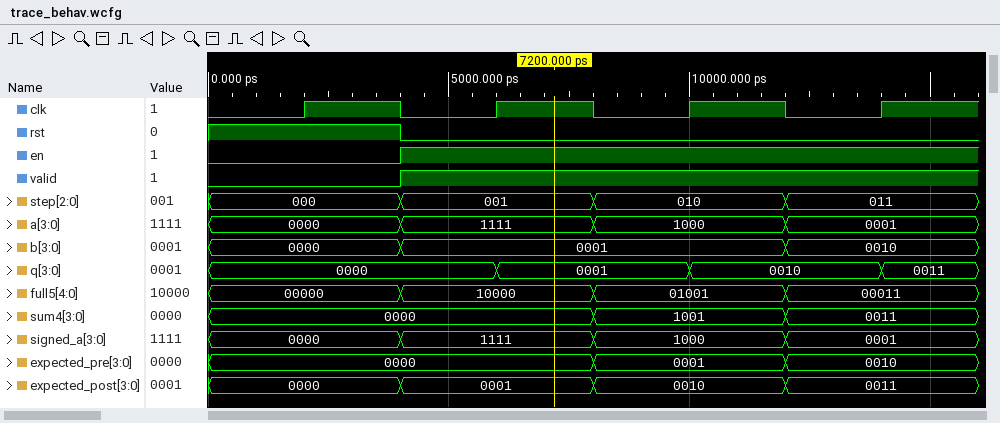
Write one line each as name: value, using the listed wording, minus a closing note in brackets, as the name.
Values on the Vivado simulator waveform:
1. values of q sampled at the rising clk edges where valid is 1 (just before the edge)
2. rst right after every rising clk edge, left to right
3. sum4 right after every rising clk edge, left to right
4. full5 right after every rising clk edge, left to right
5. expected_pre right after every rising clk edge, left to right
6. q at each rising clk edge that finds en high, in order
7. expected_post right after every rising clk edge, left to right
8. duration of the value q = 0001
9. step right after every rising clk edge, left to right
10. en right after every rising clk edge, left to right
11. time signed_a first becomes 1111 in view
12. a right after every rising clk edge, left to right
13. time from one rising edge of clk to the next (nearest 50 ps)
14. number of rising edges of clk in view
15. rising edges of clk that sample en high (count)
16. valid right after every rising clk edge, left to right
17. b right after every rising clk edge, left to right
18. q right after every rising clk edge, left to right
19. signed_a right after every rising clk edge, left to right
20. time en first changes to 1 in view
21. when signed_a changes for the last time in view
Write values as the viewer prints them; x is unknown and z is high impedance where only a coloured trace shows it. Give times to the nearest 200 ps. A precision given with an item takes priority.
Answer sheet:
values of q sampled at the rising clk edges where valid is 1: 0000, 0001, 0010
rst right after every rising clk edge, left to right: 1 0 0 0
sum4 right after every rising clk edge, left to right: 0000, 0000, 1001, 0011
full5 right after every rising clk edge, left to right: 00000, 10000, 01001, 00011
expected_pre right after every rising clk edge, left to right: 0000, 0000, 0001, 0010
q at each rising clk edge that finds en high, in order: 0000, 0001, 0010
expected_post right after every rising clk edge, left to right: 0000, 0001, 0010, 0011
duration of the value q = 0001: 4000 ps
step right after every rising clk edge, left to right: 000, 001, 010, 011
en right after every rising clk edge, left to right: 0 1 1 1
time signed_a first becomes 1111 in view: 4000 ps
a right after every rising clk edge, left to right: 0000, 1111, 1000, 0001
time from one rising edge of clk to the next: 4000 ps
number of rising edges of clk in view: 4
rising edges of clk that sample en high: 3
valid right after every rising clk edge, left to right: 0 1 1 1
b right after every rising clk edge, left to right: 0000, 0001, 0001, 0010
q right after every rising clk edge, left to right: 0000, 0001, 0010, 0011
signed_a right after every rising clk edge, left to right: 0000, 1111, 1000, 0001
time en first changes to 1 in view: 4000 ps
when signed_a changes for the last time in view: 12000 ps
